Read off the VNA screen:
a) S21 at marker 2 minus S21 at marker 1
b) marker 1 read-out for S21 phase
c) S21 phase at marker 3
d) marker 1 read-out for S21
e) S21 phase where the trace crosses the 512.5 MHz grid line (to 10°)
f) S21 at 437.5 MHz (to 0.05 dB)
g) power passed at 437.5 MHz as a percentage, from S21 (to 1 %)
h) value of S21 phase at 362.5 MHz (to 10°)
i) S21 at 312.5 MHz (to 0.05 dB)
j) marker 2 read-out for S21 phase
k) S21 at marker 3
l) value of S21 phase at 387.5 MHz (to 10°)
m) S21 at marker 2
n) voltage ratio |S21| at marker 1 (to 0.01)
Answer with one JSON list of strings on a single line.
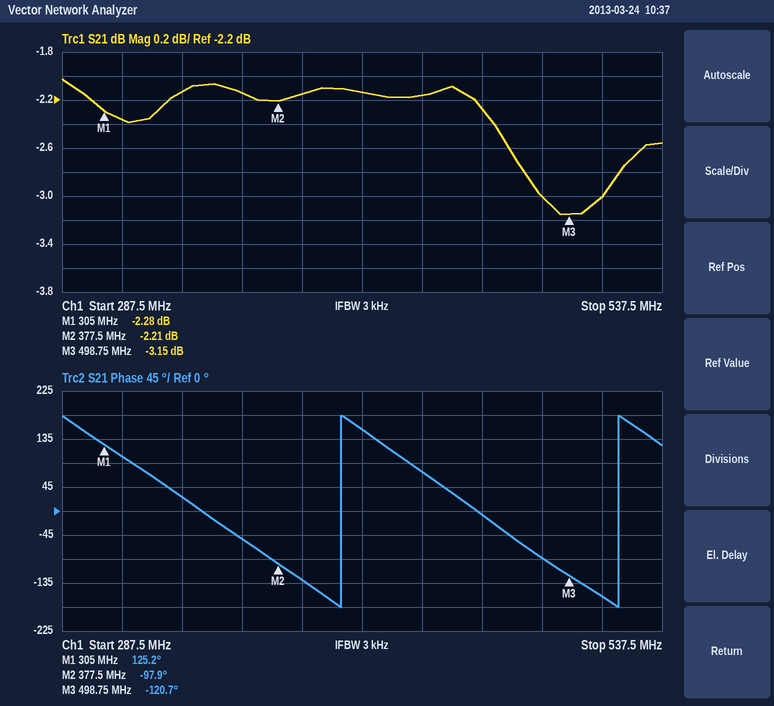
["0.07 dB", "125.2°", "-120.7°", "-2.28 dB", "-160°", "-2.15 dB", "61 %", "-50°", "-2.35 dB", "-97.9°", "-3.15 dB", "-130°", "-2.21 dB", "0.77"]
